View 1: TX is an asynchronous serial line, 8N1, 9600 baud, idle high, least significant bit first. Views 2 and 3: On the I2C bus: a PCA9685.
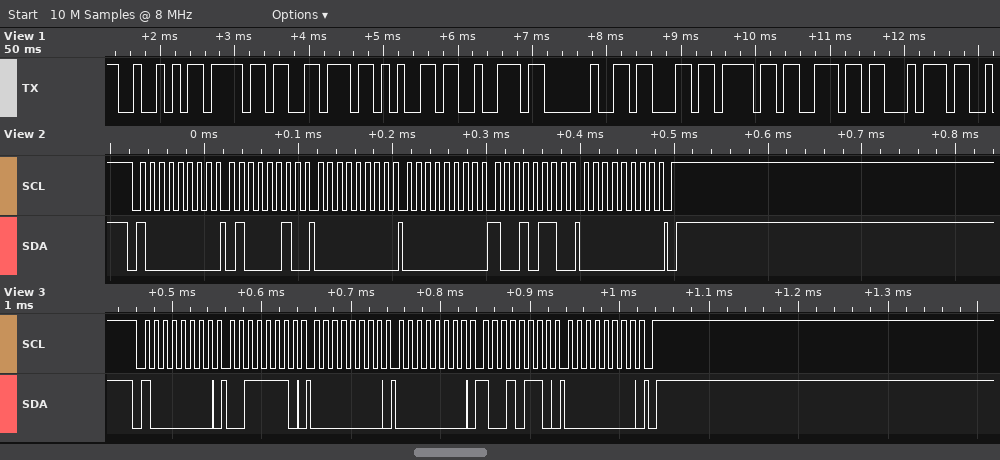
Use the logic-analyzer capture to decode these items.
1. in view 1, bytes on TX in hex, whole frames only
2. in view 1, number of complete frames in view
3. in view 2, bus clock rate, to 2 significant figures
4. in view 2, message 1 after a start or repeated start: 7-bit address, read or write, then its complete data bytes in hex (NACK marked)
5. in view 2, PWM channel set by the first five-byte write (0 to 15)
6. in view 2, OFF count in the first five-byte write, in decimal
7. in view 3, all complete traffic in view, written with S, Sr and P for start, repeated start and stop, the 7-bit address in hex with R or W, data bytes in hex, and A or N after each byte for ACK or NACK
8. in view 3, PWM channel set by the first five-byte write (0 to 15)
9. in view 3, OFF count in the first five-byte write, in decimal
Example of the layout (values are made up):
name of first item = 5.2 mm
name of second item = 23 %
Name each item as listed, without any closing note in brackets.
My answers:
in view 1, bytes on TX in hex, whole frames only = 0x52 0x6F 0x76 0x65 0x72 0x20 0x63 0x6F 0x6E 0x74
in view 1, number of complete frames in view = 10
in view 2, bus clock rate, to 2 significant figures = 100 kHz
in view 2, message 1 after a start or repeated start: 7-bit address, read or write, then its complete data bytes in hex = 0x40 write: 42 00 00 96 00
in view 2, PWM channel set by the first five-byte write = 15
in view 2, OFF count in the first five-byte write, in decimal = 150
in view 3, all complete traffic in view, written with S, Sr and P for start, repeated start and stop, the 7-bit address in hex with R or W, data bytes in hex, and A or N after each byte for ACK or NACK = S 40W A 3E A 00 A 00 A 96 A 00 A P
in view 3, PWM channel set by the first five-byte write = 14
in view 3, OFF count in the first five-byte write, in decimal = 150
